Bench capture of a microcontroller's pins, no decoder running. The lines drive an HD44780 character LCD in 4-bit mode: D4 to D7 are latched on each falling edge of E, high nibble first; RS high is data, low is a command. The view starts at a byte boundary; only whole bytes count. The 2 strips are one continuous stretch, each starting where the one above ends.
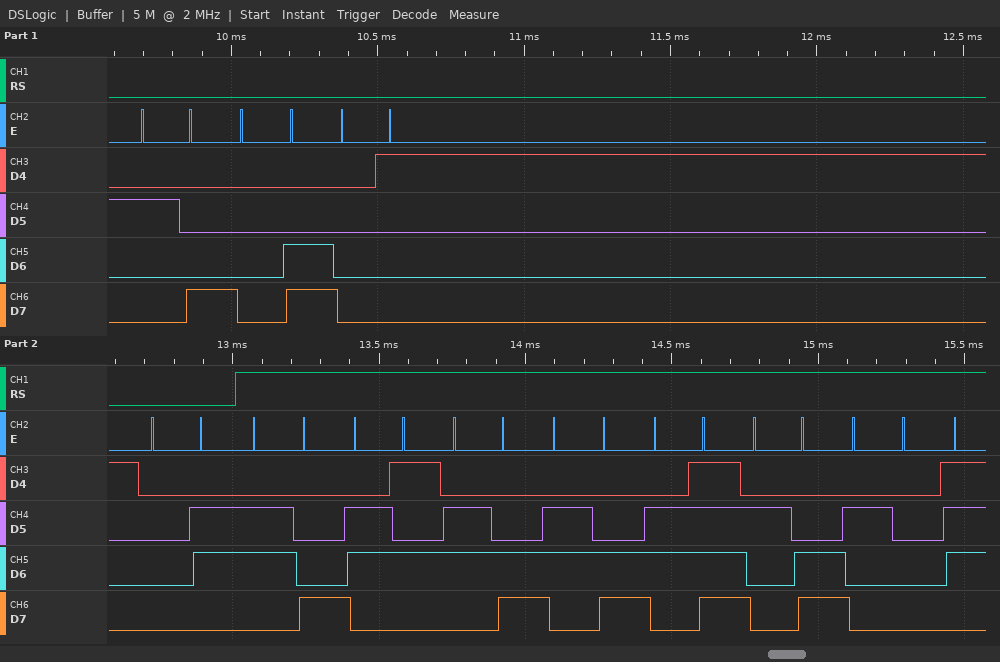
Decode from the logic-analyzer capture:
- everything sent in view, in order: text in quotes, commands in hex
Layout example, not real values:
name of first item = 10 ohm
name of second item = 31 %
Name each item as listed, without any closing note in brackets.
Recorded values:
everything sent in view, in order: text in quotes, commands in hex = 0x28 0x0C 0x01 0x06 "hello, "
